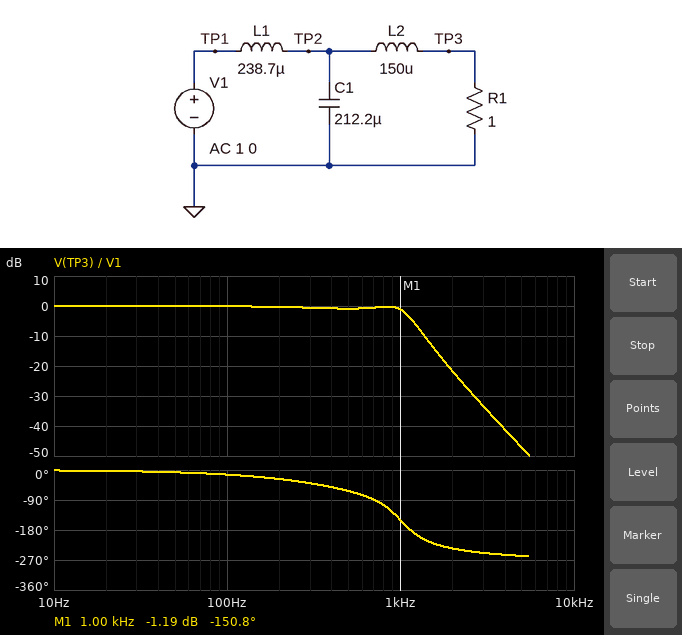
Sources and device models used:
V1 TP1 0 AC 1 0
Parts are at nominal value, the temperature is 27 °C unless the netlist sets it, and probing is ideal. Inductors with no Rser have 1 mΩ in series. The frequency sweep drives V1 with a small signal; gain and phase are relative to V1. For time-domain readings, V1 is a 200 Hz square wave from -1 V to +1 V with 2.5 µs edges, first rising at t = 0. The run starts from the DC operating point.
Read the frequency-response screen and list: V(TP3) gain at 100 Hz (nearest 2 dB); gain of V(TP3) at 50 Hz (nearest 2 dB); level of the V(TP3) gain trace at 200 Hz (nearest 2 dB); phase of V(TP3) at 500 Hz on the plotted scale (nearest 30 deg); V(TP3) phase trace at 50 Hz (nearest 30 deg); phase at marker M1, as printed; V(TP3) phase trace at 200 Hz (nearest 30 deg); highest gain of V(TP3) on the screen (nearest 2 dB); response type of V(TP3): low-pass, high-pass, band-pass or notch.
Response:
0 dB
0 dB
0 dB
-60 deg
0 deg
-150.8 deg
-30 deg
0 dB
low-pass
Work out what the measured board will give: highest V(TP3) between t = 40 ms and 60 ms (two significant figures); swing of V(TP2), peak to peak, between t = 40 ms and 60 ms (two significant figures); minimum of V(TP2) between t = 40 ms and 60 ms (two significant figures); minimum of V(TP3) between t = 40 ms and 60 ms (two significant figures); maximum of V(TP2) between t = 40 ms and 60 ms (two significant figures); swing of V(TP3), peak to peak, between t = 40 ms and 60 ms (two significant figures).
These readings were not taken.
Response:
1.1 V
2.6 V
-1.3 V
-1.1 V
1.3 V
2.3 V
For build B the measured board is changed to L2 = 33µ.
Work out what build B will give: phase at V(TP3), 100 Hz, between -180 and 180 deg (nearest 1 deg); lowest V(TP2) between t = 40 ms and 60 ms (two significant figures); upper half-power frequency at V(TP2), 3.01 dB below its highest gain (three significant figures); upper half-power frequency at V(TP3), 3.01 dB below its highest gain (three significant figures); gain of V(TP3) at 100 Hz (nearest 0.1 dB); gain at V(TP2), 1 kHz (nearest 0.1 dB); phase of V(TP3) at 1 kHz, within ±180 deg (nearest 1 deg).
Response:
-10 deg
-1.2 V
886 Hz
878 Hz
0 dB
-4.1 dB
-128 deg
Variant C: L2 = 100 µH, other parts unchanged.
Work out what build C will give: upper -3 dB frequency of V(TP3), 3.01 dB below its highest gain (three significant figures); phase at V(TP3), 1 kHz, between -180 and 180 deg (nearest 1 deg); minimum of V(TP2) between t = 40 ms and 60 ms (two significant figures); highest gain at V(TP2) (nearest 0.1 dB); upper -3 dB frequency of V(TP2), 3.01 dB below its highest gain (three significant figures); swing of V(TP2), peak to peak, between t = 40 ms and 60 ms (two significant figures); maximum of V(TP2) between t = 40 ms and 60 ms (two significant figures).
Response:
1.04 kHz
-139 deg
-1.2 V
0.3 dB
1.14 kHz
2.4 V
1.2 V
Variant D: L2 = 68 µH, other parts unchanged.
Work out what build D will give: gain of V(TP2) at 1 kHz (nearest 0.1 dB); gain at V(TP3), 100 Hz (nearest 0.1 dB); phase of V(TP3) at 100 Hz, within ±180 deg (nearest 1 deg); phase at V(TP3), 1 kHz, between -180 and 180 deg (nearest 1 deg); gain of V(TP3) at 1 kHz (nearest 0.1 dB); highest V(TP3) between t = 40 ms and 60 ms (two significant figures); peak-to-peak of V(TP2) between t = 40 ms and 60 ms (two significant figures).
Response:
-2.6 dB
0 dB
-11 deg
-133 deg
-3.3 dB
1.2 V
2.4 V
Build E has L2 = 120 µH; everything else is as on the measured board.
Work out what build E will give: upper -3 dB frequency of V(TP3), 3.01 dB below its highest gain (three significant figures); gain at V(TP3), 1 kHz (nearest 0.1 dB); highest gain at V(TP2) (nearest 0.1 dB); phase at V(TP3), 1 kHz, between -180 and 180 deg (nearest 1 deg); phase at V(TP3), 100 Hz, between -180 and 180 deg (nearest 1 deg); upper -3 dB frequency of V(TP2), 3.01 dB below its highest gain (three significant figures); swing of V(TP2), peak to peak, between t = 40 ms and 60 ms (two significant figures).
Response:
1.07 kHz
-1.9 dB
0.8 dB
-143 deg
-13 deg
1.16 kHz
2.5 V
